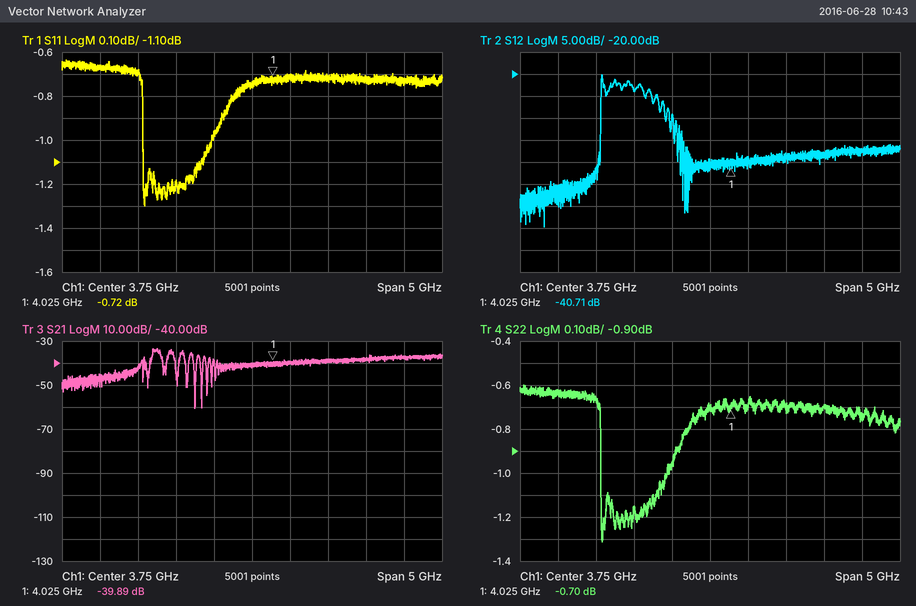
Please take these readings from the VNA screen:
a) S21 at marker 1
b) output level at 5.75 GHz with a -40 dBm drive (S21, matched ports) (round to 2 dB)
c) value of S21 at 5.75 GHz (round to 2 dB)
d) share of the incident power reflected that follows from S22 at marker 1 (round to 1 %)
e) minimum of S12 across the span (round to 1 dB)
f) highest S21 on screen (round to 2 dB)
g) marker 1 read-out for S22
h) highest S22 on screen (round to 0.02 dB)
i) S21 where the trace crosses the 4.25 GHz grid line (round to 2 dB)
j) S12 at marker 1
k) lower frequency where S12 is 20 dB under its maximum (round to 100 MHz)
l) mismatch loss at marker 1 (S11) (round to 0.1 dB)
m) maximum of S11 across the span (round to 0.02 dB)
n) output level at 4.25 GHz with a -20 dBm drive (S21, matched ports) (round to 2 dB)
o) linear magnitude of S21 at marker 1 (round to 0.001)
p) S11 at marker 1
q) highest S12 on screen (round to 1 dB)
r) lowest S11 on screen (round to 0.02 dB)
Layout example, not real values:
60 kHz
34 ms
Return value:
-39.89 dB
-78 dBm
-38 dB
85 %
-55 dB
-34 dB
-0.70 dB
-0.60 dB
-40 dB
-40.71 dB
2.3 GHz
8.2 dB
-0.64 dB
-60 dBm
0.010
-0.72 dB
-20 dB
-1.30 dB
